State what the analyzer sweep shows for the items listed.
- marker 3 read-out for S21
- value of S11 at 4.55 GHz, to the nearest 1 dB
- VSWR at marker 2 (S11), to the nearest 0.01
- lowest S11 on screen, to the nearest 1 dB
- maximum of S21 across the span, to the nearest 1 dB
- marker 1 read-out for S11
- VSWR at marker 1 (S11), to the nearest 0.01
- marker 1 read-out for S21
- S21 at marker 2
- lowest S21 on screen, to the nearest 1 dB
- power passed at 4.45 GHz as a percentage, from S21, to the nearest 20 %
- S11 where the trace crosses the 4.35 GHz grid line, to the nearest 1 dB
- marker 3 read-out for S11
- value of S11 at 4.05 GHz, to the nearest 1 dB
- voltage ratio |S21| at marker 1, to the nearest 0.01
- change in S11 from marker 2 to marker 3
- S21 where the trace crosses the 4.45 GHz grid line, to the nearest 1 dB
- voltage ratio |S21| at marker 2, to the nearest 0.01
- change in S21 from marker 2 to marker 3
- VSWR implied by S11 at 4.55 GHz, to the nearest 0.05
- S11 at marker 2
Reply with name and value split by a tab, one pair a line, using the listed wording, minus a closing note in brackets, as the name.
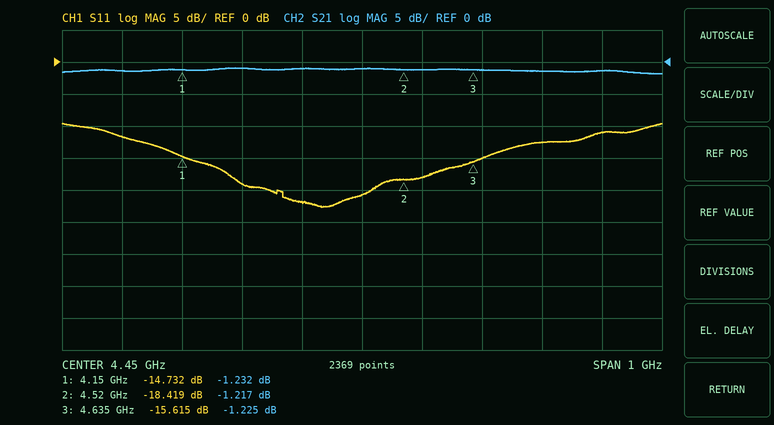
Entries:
marker 3 read-out for S21	-1.225 dB
value of S11 at 4.55 GHz, to the nearest 1 dB	-18 dB
VSWR at marker 2 (S11), to the nearest 0.01	1.27
lowest S11 on screen, to the nearest 1 dB	-23 dB
maximum of S21 across the span, to the nearest 1 dB	-1 dB
marker 1 read-out for S11	-14.732 dB
VSWR at marker 1 (S11), to the nearest 0.01	1.45
marker 1 read-out for S21	-1.232 dB
S21 at marker 2	-1.217 dB
lowest S21 on screen, to the nearest 1 dB	-2 dB
power passed at 4.45 GHz as a percentage, from S21, to the nearest 20 %	80 %
S11 where the trace crosses the 4.35 GHz grid line, to the nearest 1 dB	-22 dB
marker 3 read-out for S11	-15.615 dB
value of S11 at 4.05 GHz, to the nearest 1 dB	-12 dB
voltage ratio |S21| at marker 1, to the nearest 0.01	0.87
change in S11 from marker 2 to marker 3	2.804 dB
S21 where the trace crosses the 4.45 GHz grid line, to the nearest 1 dB	-1 dB
voltage ratio |S21| at marker 2, to the nearest 0.01	0.87
change in S21 from marker 2 to marker 3	-0.008 dB
VSWR implied by S11 at 4.55 GHz, to the nearest 0.05	1.30
S11 at marker 2	-18.419 dB
